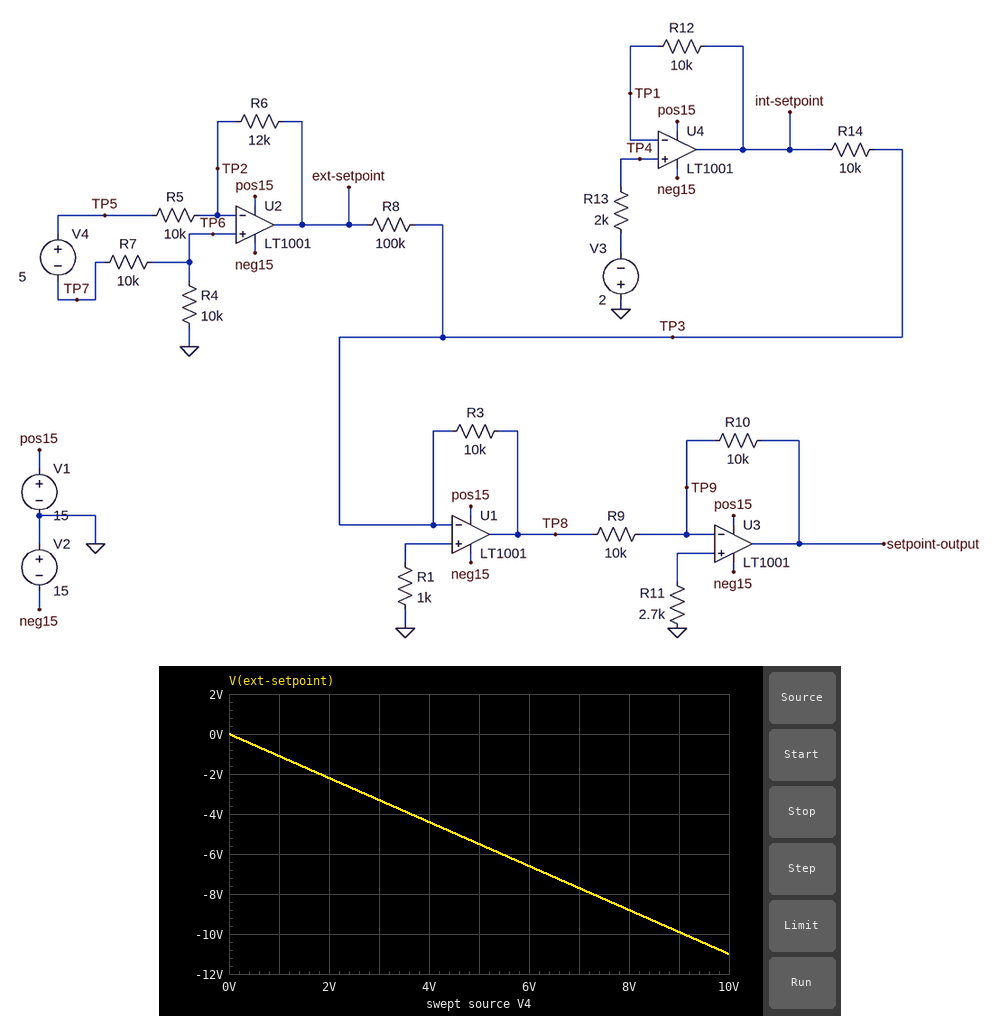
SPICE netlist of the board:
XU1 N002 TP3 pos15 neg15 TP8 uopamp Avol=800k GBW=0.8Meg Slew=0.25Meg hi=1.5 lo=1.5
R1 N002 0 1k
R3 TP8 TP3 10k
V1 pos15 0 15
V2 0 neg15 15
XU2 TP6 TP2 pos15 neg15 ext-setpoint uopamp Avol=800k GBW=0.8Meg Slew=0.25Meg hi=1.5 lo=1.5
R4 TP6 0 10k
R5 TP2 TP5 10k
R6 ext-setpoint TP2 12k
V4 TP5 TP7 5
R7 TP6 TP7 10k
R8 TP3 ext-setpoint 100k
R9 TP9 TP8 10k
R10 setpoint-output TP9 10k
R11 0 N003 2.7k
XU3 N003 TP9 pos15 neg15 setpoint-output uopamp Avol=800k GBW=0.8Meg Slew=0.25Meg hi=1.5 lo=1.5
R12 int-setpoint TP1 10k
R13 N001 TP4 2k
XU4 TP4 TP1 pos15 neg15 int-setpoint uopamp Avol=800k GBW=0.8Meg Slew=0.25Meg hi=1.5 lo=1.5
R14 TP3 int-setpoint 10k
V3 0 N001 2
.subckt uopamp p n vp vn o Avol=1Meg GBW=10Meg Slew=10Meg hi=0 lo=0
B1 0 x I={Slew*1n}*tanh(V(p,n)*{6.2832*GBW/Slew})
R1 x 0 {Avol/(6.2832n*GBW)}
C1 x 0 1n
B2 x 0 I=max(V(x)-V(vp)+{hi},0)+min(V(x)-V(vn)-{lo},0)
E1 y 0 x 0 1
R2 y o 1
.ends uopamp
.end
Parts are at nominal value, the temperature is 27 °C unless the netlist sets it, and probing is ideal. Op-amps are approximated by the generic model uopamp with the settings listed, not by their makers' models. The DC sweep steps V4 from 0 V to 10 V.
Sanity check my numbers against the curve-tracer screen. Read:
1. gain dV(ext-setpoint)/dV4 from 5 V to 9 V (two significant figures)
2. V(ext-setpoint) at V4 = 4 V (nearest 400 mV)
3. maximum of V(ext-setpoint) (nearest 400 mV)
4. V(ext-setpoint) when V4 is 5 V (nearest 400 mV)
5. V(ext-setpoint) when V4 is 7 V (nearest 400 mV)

-1.1 V/V
-4.4 V
0 V
-5.6 V
-7.6 V
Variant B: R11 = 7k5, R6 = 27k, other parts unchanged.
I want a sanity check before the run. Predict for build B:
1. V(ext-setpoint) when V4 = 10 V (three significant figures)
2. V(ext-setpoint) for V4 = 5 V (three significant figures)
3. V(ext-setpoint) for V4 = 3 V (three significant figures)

-13.5 V
-9.25 V
-5.55 V
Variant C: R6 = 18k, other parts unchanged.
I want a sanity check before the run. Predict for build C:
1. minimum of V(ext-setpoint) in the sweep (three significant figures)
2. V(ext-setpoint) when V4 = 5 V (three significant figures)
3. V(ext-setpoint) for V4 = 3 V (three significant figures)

-13.5 V
-7.00 V
-4.20 V
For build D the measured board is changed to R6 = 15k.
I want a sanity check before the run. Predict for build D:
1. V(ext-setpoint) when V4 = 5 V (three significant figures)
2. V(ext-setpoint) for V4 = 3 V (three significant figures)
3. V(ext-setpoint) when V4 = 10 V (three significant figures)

-6.25 V
-3.75 V
-12.5 V
